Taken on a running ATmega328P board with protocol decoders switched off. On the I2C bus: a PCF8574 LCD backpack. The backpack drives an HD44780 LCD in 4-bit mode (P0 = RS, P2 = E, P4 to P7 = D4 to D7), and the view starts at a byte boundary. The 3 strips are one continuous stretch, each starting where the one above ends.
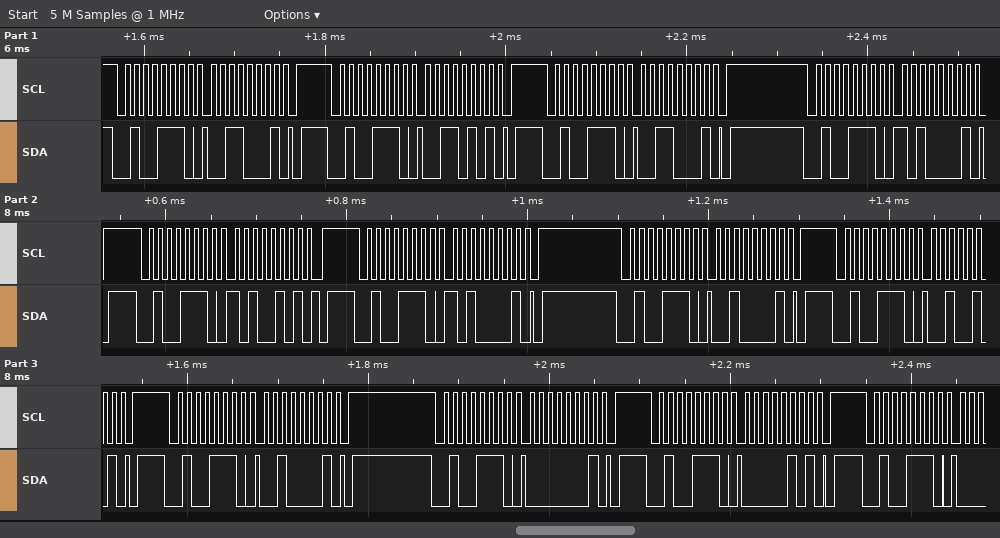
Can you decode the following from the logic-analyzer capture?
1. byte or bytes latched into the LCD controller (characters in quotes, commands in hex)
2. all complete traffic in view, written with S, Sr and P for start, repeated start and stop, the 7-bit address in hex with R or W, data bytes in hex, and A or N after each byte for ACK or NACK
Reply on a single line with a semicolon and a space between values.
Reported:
':'; S 27W A 31 A P S 27W A 35 A P S 27W A 31 A P S 27W A A1 A P S 27W A A5 A P S 27W A A1 A P S 27W A 21 A P S 27W A 25 A P S 27W A 21 A P S 27W A 01 A P S 27W A 05 A P S 27W A
